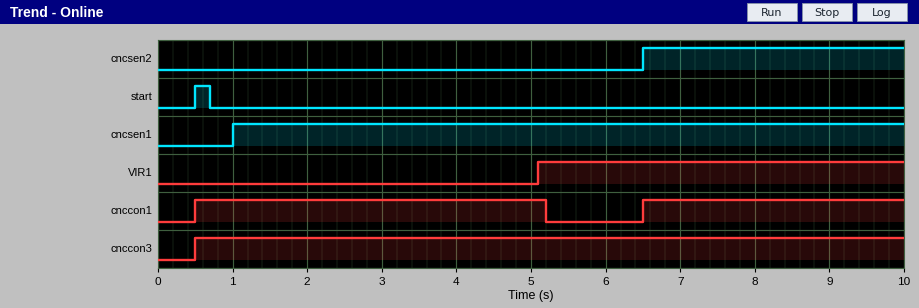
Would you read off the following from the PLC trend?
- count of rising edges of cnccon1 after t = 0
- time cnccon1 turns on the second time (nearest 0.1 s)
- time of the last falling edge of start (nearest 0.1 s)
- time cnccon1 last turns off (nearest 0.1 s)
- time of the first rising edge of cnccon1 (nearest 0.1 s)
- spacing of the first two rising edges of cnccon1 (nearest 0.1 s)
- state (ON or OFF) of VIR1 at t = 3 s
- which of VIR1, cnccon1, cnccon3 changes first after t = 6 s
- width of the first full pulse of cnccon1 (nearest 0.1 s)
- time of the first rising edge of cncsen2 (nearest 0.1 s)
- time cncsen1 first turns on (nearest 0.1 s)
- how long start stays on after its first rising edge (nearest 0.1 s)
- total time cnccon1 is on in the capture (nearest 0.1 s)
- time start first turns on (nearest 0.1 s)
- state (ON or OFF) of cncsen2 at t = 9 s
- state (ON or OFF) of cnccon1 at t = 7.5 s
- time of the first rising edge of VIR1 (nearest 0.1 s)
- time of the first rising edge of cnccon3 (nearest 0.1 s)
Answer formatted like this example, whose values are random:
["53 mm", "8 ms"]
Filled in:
["2", "6.5 s", "0.7 s", "5.2 s", "0.5 s", "6.0 s", "OFF", "cnccon1", "4.7 s", "6.5 s", "1.0 s", "0.2 s", "8.2 s", "0.5 s", "ON", "ON", "5.1 s", "0.5 s"]
